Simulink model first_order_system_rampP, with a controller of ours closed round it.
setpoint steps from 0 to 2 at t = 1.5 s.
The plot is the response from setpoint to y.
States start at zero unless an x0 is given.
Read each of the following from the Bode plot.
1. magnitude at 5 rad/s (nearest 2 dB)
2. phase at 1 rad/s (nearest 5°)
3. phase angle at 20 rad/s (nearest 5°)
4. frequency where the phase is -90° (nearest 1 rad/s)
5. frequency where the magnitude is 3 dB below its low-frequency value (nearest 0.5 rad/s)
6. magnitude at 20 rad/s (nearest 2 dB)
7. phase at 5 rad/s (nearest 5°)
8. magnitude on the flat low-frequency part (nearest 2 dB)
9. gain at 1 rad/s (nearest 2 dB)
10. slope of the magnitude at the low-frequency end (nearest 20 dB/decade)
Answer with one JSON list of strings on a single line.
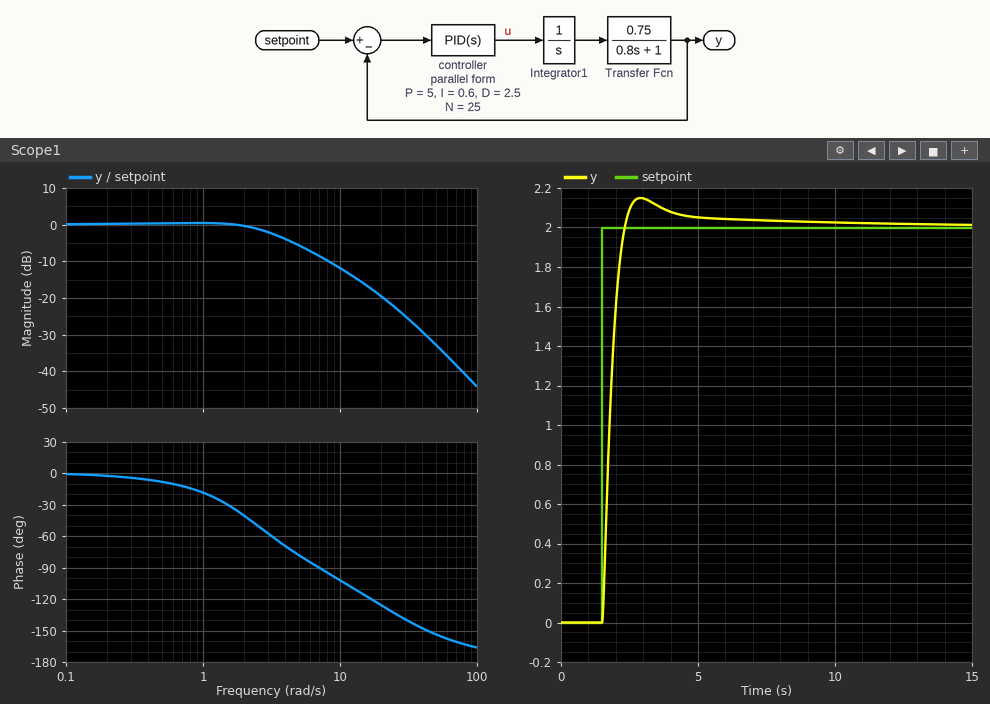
["-6 dB", "-20°", "-125°", "7 rad/s", "3.5 rad/s", "-20 dB", "-80°", "0 dB", "0 dB", "0 dB/decade"]
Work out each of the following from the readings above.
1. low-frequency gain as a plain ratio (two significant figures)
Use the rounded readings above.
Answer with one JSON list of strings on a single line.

["1.0"]
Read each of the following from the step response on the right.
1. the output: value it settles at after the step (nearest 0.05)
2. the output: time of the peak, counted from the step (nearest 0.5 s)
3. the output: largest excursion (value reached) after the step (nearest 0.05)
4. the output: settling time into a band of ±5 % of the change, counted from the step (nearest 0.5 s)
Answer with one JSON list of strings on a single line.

["2.00", "1.5 s", "2.15", "2.0 s"]
